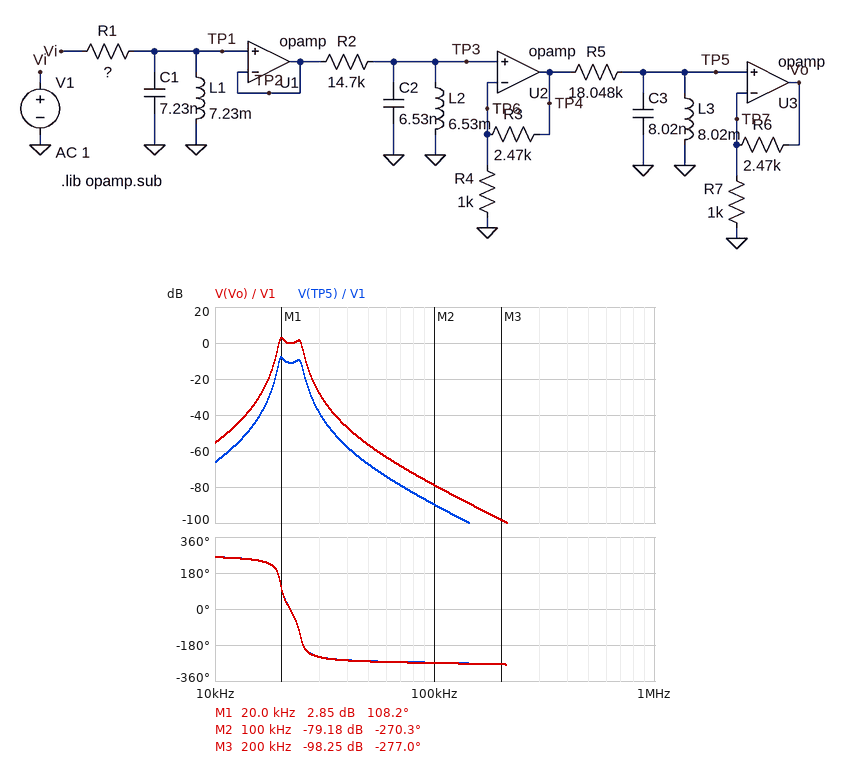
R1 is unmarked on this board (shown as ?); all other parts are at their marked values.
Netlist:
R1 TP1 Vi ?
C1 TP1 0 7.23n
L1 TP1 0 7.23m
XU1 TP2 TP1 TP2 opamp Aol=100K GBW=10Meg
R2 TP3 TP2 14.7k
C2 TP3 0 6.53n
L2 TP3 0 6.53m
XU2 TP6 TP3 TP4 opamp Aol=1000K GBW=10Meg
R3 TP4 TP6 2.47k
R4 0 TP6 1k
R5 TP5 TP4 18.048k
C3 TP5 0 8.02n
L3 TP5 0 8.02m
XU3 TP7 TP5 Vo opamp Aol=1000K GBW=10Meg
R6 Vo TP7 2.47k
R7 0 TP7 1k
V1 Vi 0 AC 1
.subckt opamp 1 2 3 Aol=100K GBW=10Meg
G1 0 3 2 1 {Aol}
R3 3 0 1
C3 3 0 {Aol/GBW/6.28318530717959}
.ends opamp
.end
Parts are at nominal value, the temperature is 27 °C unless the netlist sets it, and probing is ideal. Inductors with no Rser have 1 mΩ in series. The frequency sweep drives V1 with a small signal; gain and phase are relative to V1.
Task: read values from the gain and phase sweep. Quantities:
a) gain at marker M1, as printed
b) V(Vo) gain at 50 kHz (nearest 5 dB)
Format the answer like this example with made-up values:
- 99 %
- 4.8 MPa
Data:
- 2.85 dB
- -55 dB
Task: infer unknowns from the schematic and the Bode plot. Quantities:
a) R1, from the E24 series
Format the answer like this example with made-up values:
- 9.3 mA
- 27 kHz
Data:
- 5.1 kΩ
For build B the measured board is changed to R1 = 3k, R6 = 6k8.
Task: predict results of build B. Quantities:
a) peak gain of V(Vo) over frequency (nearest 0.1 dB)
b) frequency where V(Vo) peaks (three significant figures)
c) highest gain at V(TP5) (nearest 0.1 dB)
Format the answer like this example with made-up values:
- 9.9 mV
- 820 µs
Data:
- 11.6 dB
- 20.0 kHz
- -6.2 dB
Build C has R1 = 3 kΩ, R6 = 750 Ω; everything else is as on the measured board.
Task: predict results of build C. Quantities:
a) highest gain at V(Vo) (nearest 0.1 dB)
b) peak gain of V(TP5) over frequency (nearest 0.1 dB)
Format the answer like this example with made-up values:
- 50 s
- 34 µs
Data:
- -1.4 dB
- -6.2 dB
